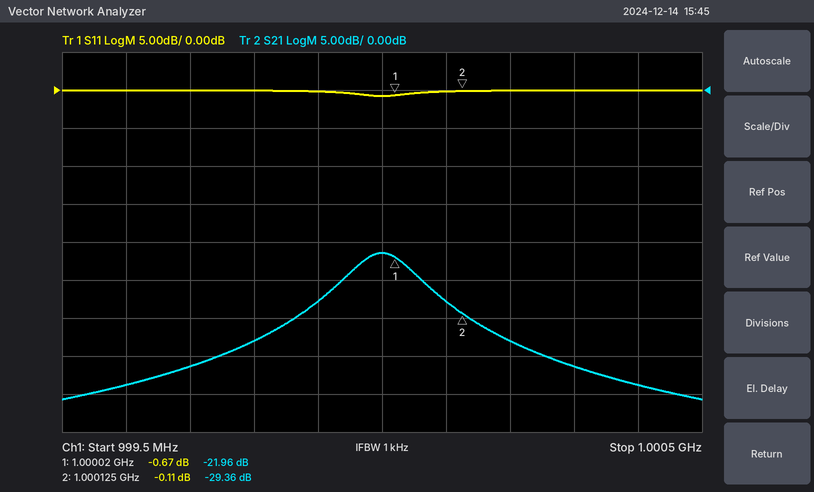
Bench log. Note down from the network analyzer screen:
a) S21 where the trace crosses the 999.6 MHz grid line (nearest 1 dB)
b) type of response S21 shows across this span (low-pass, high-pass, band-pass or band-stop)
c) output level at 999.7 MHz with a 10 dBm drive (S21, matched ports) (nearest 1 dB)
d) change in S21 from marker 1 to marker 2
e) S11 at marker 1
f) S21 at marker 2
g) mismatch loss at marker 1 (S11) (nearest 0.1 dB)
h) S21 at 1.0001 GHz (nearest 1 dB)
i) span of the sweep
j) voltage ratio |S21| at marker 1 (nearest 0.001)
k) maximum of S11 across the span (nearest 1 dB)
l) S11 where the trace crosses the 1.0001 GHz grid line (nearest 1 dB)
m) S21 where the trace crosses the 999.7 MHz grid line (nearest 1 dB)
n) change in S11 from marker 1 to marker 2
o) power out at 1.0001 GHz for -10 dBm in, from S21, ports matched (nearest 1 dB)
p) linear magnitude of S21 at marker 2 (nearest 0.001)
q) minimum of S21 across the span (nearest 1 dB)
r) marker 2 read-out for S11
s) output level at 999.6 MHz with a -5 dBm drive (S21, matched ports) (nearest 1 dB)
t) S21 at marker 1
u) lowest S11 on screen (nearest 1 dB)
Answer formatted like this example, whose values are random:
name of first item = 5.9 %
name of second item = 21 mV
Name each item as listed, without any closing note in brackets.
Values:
S21 where the trace crosses the 999.6 MHz grid line = -39 dB
type of response S21 shows across this span = band-pass
output level at 999.7 MHz with a 10 dBm drive (S21, matched ports) = -26 dBm
change in S21 from marker 1 to marker 2 = -7.40 dB
S11 at marker 1 = -0.67 dB
S21 at marker 2 = -29.36 dB
mismatch loss at marker 1 (S11) = 8.4 dB
S21 at 1.0001 GHz = -28 dB
span of the sweep = 1 MHz
voltage ratio |S21| at marker 1 = 0.080
maximum of S11 across the span = 0 dB
S11 where the trace crosses the 1.0001 GHz grid line = 0 dB
S21 where the trace crosses the 999.7 MHz grid line = -36 dB
change in S11 from marker 1 to marker 2 = 0.56 dB
power out at 1.0001 GHz for -10 dBm in, from S21, ports matched = -38 dBm
linear magnitude of S21 at marker 2 = 0.034
minimum of S21 across the span = -41 dB
marker 2 read-out for S11 = -0.11 dB
output level at 999.6 MHz with a -5 dBm drive (S21, matched ports) = -44 dBm
S21 at marker 1 = -21.96 dB
lowest S11 on screen = -1 dB
